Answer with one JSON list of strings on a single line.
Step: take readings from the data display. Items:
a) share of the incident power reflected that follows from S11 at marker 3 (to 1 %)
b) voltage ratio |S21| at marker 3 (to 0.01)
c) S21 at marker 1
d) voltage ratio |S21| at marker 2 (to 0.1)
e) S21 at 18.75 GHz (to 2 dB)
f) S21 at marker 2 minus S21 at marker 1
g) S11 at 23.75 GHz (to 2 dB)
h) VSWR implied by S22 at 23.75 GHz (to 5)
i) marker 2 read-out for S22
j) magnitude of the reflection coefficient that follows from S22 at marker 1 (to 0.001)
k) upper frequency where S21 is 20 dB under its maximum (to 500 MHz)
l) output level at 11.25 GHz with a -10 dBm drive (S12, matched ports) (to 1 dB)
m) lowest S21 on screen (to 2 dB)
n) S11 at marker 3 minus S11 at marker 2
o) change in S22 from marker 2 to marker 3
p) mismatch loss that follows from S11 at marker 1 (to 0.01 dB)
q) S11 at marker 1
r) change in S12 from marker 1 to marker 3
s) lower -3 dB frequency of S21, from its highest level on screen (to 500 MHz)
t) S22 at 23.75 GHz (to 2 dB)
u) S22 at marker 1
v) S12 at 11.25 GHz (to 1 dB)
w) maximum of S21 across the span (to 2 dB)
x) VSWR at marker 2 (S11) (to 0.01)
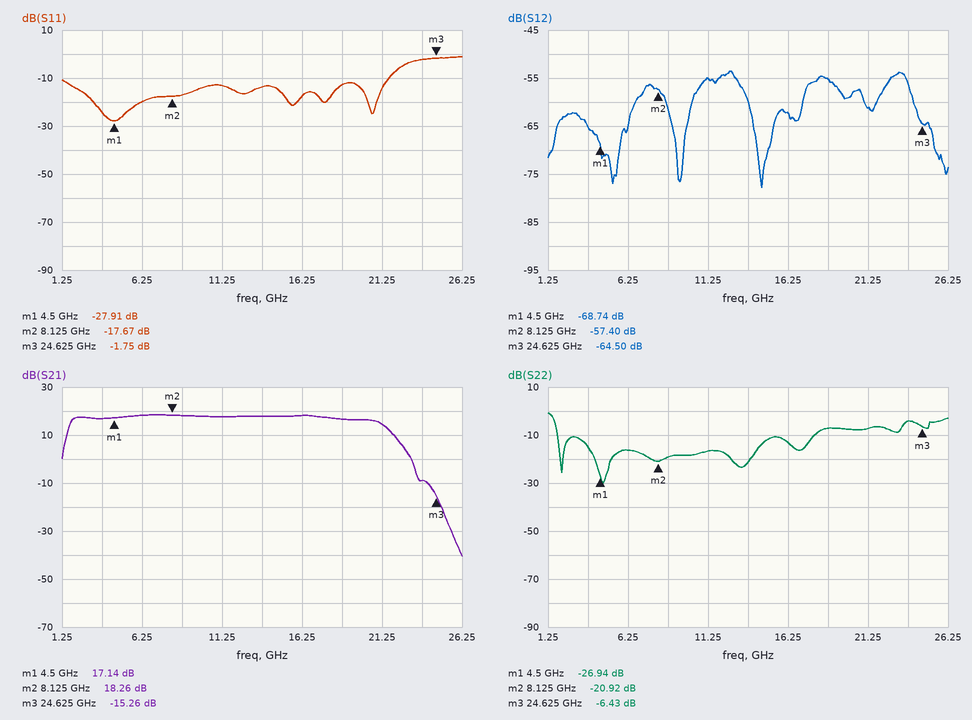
["67 %", "0.17", "17.14 dB", "8.2", "16 dB", "1.12 dB", "-2 dB", "5", "-20.92 dB", "0.045", "23.0 GHz", "-65 dBm", "-40 dB", "15.92 dB", "14.49 dB", "0.01 dB", "-27.91 dB", "4.24 dB", "2.0 GHz", "-4 dB", "-26.94 dB", "-55 dB", "18 dB", "1.30"]
